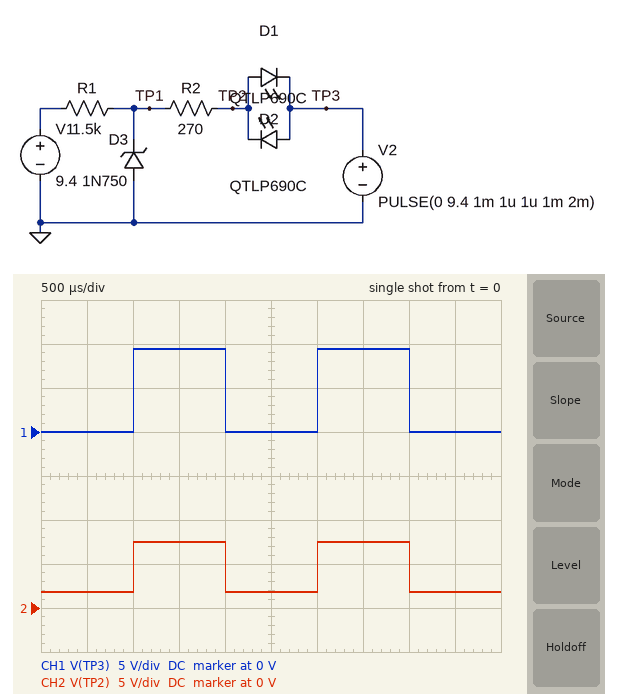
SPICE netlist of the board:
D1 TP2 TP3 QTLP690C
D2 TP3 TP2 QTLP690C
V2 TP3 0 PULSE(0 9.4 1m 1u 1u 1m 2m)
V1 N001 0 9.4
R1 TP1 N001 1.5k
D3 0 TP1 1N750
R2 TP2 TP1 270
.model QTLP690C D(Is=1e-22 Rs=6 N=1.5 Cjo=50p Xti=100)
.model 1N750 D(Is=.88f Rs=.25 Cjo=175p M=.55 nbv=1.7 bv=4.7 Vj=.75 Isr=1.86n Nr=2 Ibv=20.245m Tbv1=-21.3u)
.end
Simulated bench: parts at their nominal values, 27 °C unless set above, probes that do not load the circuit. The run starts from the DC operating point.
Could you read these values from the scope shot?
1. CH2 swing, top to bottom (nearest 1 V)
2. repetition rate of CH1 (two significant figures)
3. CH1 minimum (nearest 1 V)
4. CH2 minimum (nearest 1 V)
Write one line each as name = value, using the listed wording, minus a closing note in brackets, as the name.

CH2 swing, top to bottom = 6 V
repetition rate of CH1 = 500 Hz
CH1 minimum = 0 V
CH2 minimum = 2 V
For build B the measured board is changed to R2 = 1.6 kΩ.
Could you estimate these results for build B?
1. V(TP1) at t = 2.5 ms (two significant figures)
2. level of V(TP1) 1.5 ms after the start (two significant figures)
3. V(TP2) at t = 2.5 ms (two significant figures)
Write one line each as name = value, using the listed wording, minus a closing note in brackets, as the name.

V(TP1) at t = 2.5 ms = 4.6 V
level of V(TP1) 1.5 ms after the start = 4.6 V
V(TP2) at t = 2.5 ms = 1.7 V
